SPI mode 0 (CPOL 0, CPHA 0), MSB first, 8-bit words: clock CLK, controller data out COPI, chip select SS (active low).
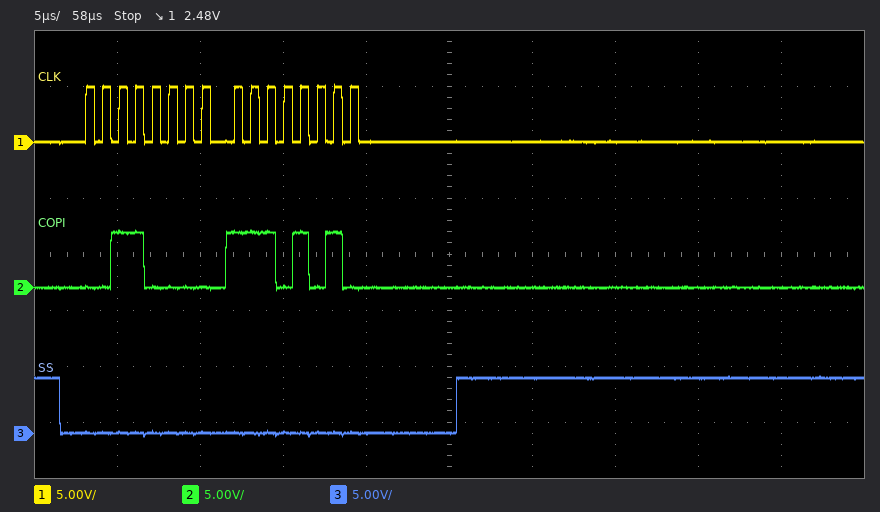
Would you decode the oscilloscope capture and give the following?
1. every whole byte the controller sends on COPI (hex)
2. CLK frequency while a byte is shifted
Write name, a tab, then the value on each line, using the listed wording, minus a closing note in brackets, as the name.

every whole byte the controller sends on COPI	30 EA
CLK frequency while a byte is shifted	1 MHz
